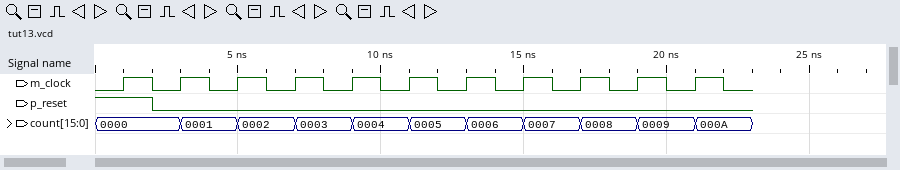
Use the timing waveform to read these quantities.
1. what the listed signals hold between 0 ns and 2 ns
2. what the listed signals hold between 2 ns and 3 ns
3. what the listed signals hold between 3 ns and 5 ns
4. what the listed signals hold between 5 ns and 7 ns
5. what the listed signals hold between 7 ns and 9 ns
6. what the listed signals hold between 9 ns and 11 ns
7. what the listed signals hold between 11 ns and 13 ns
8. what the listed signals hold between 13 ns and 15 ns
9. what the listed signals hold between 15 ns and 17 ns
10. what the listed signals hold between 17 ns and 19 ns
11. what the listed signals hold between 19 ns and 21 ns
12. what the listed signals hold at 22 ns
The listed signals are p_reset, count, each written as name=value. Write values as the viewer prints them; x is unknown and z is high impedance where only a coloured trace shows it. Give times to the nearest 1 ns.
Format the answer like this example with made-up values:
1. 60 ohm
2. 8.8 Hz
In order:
1. p_reset=1, count=0000
2. p_reset=0, count=0000
3. p_reset=0, count=0001
4. p_reset=0, count=0002
5. p_reset=0, count=0003
6. p_reset=0, count=0004
7. p_reset=0, count=0005
8. p_reset=0, count=0006
9. p_reset=0, count=0007
10. p_reset=0, count=0008
11. p_reset=0, count=0009
12. p_reset=0, count=000A
